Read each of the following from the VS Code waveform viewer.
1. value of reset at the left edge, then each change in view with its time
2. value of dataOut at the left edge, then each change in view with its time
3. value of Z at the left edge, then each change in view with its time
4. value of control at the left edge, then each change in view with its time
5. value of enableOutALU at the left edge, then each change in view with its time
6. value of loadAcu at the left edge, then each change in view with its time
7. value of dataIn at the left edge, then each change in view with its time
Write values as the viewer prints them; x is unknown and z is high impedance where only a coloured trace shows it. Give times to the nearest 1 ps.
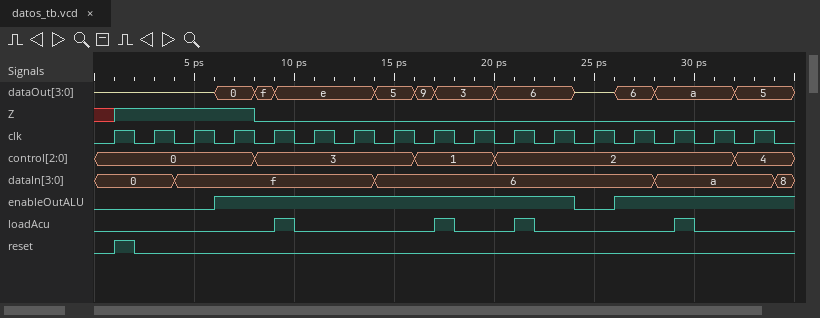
0, 1 at 1 ps, 0 at 2 ps
z, 0 at 6 ps, f at 8 ps, e at 9 ps, 5 at 14 ps, 9 at 16 ps, 3 at 17 ps, 6 at 20 ps, z at 24 ps, 6 at 26 ps, a at 28 ps, 5 at 32 ps
x, 1 at 1 ps, 0 at 8 ps
0, 3 at 8 ps, 1 at 16 ps, 2 at 20 ps, 4 at 32 ps
0, 1 at 6 ps, 0 at 24 ps, 1 at 26 ps
0, 1 at 9 ps, 0 at 10 ps, 1 at 17 ps, 0 at 18 ps, 1 at 21 ps, 0 at 22 ps, 1 at 29 ps, 0 at 30 ps
0, f at 4 ps, 6 at 14 ps, a at 28 ps, 8 at 34 ps
